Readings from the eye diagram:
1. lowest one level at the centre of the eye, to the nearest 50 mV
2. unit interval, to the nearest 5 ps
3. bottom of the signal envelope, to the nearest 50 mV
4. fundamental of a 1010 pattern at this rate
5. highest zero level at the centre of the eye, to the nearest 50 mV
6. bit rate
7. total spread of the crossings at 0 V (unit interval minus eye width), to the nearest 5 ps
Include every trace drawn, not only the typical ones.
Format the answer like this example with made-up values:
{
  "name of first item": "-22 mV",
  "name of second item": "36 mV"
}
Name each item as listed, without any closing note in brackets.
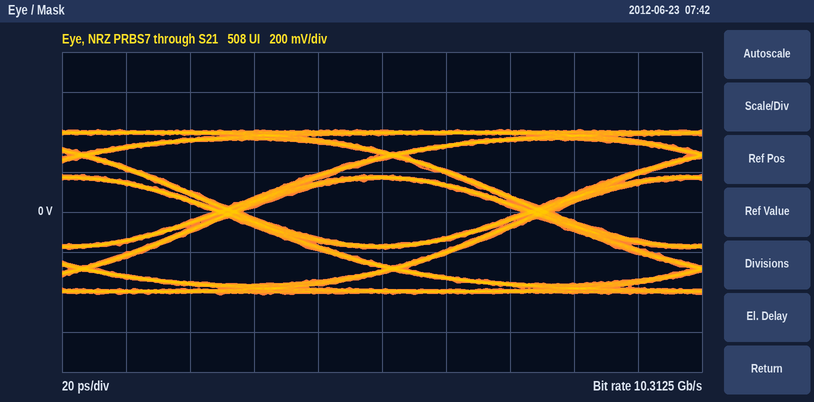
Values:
{
  "lowest one level at the centre of the eye, to the nearest 50 mV": "150 mV",
  "unit interval, to the nearest 5 ps": "95 ps",
  "bottom of the signal envelope, to the nearest 50 mV": "-400 mV",
  "fundamental of a 1010 pattern at this rate": "5.15625 GHz",
  "highest zero level at the centre of the eye, to the nearest 50 mV": "-150 mV",
  "bit rate": "10.3125 Gb/s",
  "total spread of the crossings at 0 V (unit interval minus eye width), to the nearest 5 ps": "10 ps"
}
